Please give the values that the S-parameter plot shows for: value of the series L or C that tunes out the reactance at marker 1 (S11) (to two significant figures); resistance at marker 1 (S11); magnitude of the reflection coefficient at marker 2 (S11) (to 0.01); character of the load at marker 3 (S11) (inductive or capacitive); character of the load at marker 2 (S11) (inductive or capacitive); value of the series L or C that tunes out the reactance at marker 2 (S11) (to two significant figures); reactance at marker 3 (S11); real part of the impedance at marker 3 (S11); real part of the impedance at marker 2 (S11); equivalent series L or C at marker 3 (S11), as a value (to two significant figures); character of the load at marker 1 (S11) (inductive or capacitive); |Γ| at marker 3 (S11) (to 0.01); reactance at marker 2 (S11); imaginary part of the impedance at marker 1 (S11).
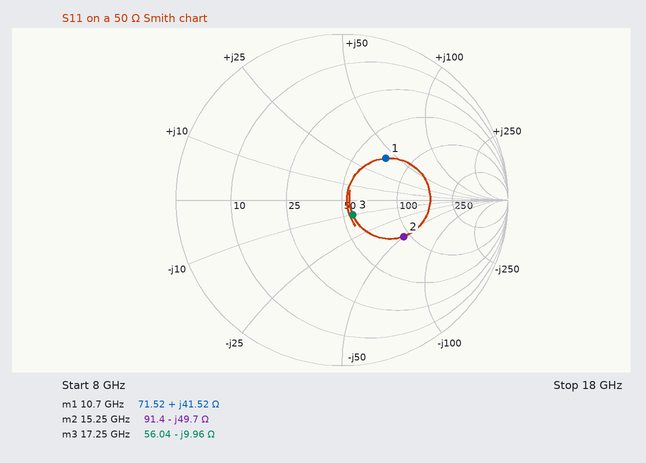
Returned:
360 fF
71.52 Ω
0.43
capacitive
capacitive
520 pH
-9.96 Ω
56.04 Ω
91.4 Ω
930 fF
inductive
0.11
-49.7 Ω
+41.52 Ω
